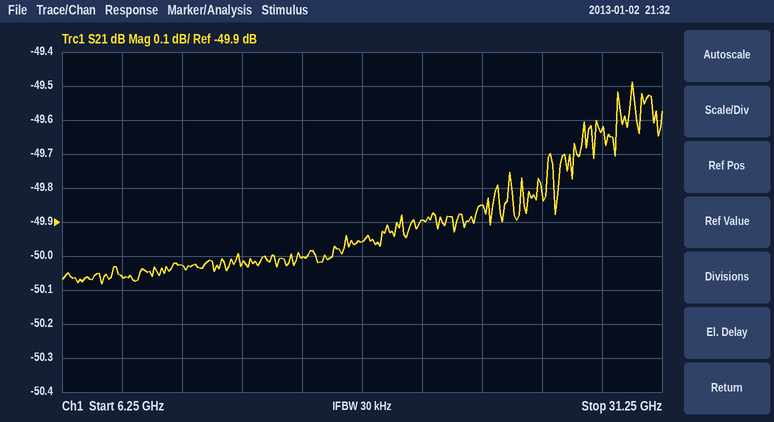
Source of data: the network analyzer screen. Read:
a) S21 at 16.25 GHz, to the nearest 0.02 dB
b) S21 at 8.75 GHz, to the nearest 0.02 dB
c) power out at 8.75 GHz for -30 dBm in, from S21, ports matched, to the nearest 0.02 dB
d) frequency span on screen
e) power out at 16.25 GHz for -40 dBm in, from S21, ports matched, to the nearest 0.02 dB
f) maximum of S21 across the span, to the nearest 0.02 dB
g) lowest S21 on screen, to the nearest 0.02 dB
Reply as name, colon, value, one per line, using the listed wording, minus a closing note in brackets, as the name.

S21 at 16.25 GHz, to the nearest 0.02 dB: -50.00 dB
S21 at 8.75 GHz, to the nearest 0.02 dB: -50.06 dB
power out at 8.75 GHz for -30 dBm in, from S21, ports matched, to the nearest 0.02 dB: -80.06 dBm
frequency span on screen: 25 GHz
power out at 16.25 GHz for -40 dBm in, from S21, ports matched, to the nearest 0.02 dB: -90.00 dBm
maximum of S21 across the span, to the nearest 0.02 dB: -49.48 dB
lowest S21 on screen, to the nearest 0.02 dB: -50.08 dB
